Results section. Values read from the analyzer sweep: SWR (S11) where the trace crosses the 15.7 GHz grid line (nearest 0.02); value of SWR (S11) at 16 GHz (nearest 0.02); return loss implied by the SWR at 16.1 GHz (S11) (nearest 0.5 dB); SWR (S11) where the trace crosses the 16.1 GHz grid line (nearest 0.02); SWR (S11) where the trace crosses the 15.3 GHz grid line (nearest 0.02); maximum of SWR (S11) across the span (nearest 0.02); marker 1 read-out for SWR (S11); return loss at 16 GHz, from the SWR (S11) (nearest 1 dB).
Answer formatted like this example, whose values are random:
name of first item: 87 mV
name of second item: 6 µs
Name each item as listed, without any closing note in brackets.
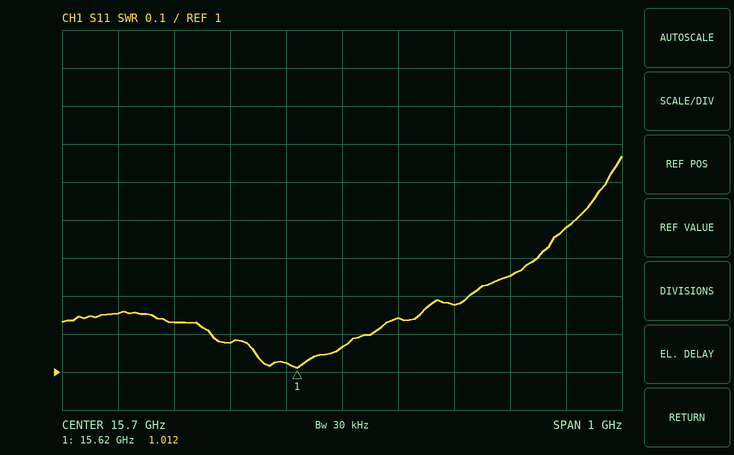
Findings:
SWR (S11) where the trace crosses the 15.7 GHz grid line: 1.06
value of SWR (S11) at 16 GHz: 1.26
return loss implied by the SWR at 16.1 GHz (S11): 16.0 dB
SWR (S11) where the trace crosses the 16.1 GHz grid line: 1.38
SWR (S11) where the trace crosses the 15.3 GHz grid line: 1.16
maximum of SWR (S11) across the span: 1.56
marker 1 read-out for SWR: 1.012
return loss at 16 GHz, from the SWR (S11): 19 dB
